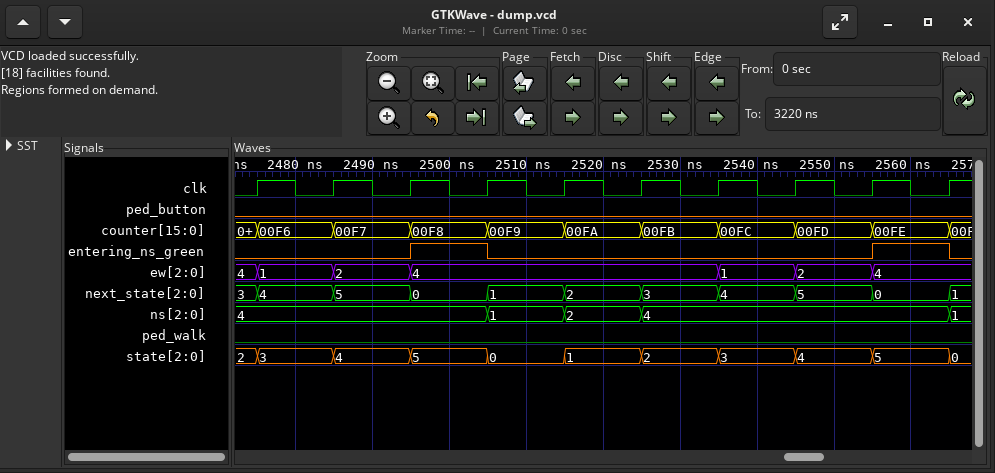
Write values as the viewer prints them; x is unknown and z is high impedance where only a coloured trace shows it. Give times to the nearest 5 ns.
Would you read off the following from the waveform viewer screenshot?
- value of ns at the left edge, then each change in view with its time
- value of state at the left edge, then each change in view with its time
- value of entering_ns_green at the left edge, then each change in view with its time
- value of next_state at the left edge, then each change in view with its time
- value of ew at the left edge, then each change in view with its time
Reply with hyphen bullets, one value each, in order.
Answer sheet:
- 4, 1 at 2505 ns, 2 at 2515 ns, 4 at 2525 ns, 1 at 2565 ns
- 2, 3 at 2475 ns, 4 at 2485 ns, 5 at 2495 ns, 0 at 2505 ns, 1 at 2515 ns, 2 at 2525 ns, 3 at 2535 ns, 4 at 2545 ns, 5 at 2555 ns, 0 at 2565 ns
- 0, 1 at 2495 ns, 0 at 2505 ns, 1 at 2555 ns, 0 at 2565 ns
- 3, 4 at 2475 ns, 5 at 2485 ns, 0 at 2495 ns, 1 at 2505 ns, 2 at 2515 ns, 3 at 2525 ns, 4 at 2535 ns, 5 at 2545 ns, 0 at 2555 ns, 1 at 2565 ns
- 4, 1 at 2475 ns, 2 at 2485 ns, 4 at 2495 ns, 1 at 2535 ns, 2 at 2545 ns, 4 at 2555 ns
